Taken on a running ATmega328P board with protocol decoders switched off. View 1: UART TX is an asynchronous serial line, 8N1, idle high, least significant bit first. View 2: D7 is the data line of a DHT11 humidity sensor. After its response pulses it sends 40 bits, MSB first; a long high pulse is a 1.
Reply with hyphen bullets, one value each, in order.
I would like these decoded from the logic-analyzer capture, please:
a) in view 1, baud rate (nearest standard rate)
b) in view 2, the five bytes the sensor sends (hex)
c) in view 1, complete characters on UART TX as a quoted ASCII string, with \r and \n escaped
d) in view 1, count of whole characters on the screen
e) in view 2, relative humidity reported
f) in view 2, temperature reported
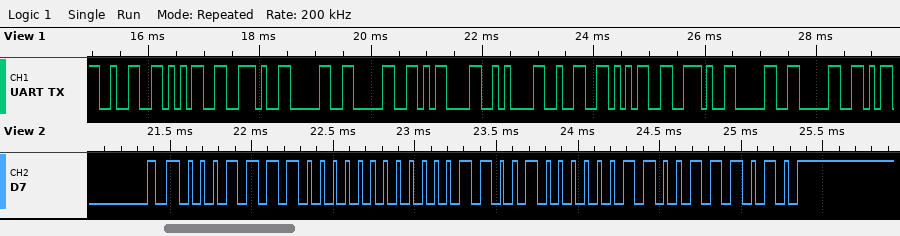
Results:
- 9600 baud
- 1E 00 19 03 3A
- "25.00\r\n25.00"
- 12
- 30 %
- 25.3 °C
